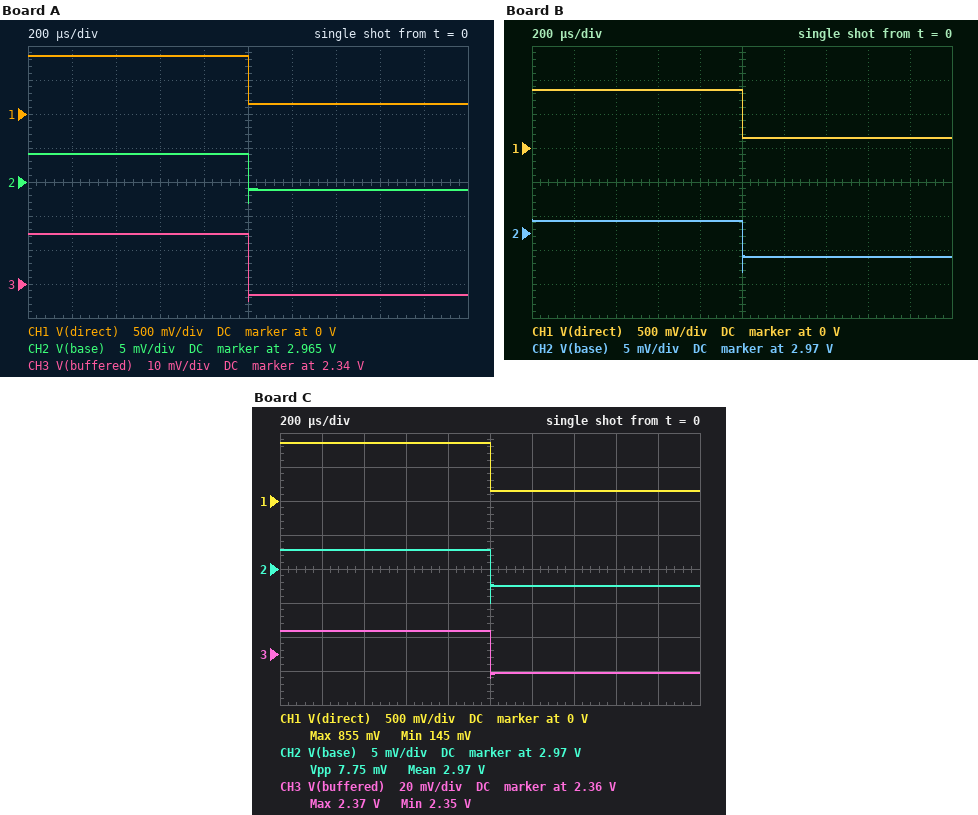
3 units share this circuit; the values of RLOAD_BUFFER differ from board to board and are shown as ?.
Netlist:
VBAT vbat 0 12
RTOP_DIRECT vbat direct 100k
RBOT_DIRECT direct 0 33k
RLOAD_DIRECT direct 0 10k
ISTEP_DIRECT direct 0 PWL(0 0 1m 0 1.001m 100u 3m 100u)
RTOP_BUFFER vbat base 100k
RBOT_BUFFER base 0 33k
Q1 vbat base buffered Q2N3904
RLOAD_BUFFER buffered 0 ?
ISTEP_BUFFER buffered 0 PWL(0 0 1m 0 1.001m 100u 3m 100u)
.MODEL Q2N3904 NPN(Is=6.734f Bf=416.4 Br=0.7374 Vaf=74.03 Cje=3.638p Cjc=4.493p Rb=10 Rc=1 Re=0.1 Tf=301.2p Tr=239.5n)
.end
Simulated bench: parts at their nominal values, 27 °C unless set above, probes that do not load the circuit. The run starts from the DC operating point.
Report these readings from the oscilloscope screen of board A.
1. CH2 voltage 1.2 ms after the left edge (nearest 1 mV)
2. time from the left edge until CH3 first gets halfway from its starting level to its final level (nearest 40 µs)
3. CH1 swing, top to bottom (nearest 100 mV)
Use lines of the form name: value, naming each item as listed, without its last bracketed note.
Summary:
CH2 voltage 1.2 ms after the left edge: 2.964 V
time from the left edge until CH3 first gets halfway from its starting level to its final level: 1.00 ms
CH1 swing, top to bottom: 700 mV
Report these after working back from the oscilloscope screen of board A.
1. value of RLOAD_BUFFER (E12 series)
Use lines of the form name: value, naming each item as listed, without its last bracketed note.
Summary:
value of RLOAD_BUFFER: 15 kΩ
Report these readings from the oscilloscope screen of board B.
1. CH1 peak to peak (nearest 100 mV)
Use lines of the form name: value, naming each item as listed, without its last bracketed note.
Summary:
CH1 peak to peak: 700 mV
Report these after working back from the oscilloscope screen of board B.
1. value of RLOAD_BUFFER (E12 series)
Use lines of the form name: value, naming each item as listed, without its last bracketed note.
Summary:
value of RLOAD_BUFFER: 22 kΩ
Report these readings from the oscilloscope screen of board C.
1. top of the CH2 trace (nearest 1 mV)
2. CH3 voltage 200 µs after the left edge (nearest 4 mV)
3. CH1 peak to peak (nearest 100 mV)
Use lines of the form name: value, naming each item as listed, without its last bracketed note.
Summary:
top of the CH2 trace: 2.973 V
CH3 voltage 200 µs after the left edge: 2.372 V
CH1 peak to peak: 700 mV
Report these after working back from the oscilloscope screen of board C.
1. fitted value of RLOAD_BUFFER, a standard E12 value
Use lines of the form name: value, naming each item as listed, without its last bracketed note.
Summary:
fitted value of RLOAD_BUFFER, a standard E12 value: 27 kΩ
